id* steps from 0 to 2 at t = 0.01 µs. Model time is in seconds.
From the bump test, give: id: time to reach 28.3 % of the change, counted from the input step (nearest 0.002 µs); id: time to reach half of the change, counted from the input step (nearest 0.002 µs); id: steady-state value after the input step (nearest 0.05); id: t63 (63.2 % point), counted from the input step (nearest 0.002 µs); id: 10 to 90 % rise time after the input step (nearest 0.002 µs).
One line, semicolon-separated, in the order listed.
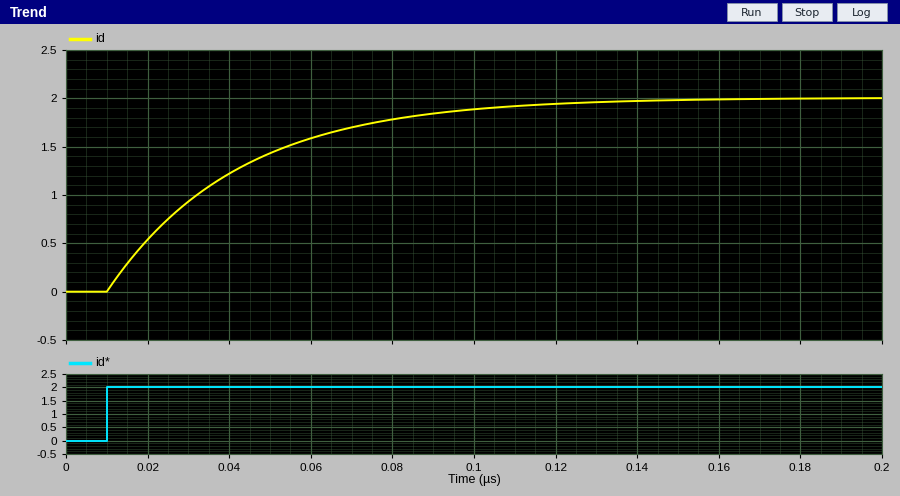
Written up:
0.010 µs; 0.022 µs; 2.00; 0.032 µs; 0.070 µs
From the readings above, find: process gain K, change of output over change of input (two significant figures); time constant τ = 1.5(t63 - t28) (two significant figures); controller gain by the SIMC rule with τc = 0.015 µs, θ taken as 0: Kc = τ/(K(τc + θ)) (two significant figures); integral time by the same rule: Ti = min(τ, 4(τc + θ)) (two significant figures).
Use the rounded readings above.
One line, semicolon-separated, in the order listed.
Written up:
1.0; 0.033 µs; 2.2; 0.033 µs
